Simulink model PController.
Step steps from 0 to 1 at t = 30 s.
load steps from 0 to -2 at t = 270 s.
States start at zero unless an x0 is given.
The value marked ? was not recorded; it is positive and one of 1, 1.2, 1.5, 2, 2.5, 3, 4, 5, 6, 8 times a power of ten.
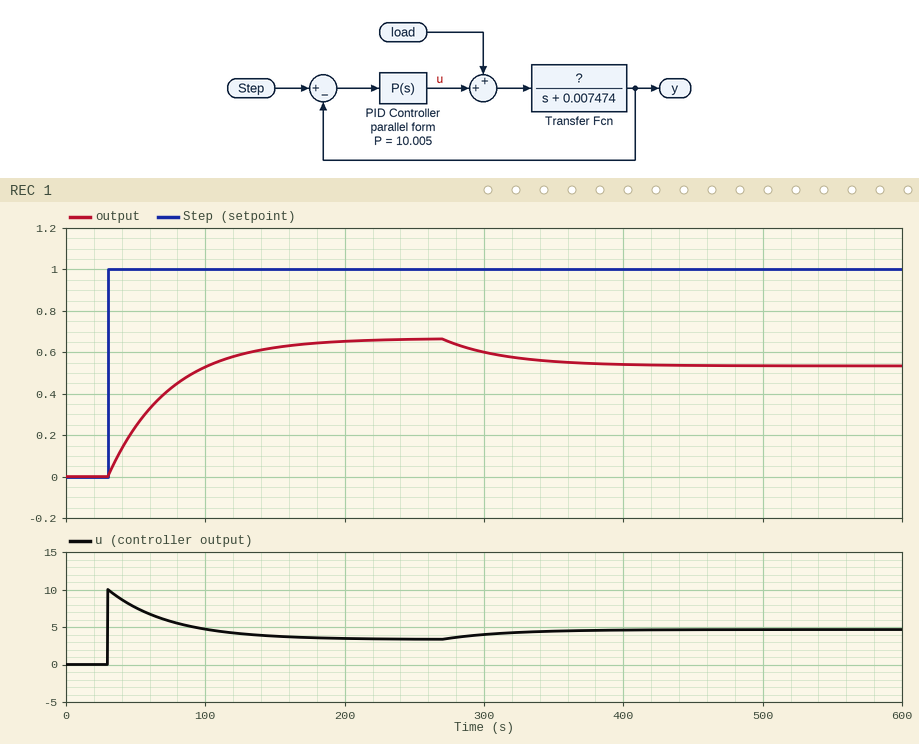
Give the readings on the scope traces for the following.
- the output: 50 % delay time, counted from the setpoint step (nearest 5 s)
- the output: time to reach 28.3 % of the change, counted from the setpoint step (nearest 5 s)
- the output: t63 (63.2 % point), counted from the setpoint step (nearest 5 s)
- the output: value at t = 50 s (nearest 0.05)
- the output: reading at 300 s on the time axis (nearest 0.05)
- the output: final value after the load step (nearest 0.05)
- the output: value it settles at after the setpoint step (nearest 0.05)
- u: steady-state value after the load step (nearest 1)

30 s
15 s
45 s
0.25
0.60
0.55
0.65
5
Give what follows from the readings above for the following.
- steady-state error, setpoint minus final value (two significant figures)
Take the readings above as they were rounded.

0.35
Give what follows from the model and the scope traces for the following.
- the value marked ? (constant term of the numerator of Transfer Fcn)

0.0015
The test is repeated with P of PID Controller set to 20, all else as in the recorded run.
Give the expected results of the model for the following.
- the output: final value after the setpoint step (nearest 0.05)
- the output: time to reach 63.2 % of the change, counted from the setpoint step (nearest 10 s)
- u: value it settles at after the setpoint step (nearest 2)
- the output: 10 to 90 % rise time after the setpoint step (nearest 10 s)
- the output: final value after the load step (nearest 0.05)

0.80
30 s
4
60 s
0.70
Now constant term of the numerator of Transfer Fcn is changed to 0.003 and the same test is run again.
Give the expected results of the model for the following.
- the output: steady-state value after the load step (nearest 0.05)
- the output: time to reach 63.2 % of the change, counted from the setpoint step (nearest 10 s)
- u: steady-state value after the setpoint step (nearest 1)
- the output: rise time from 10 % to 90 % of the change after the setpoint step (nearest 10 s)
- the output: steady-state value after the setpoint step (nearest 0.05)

0.65
30 s
2
60 s
0.80
